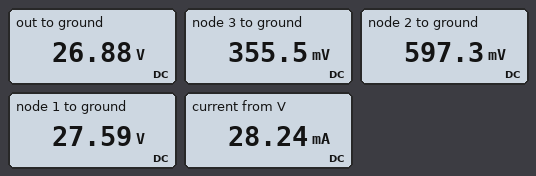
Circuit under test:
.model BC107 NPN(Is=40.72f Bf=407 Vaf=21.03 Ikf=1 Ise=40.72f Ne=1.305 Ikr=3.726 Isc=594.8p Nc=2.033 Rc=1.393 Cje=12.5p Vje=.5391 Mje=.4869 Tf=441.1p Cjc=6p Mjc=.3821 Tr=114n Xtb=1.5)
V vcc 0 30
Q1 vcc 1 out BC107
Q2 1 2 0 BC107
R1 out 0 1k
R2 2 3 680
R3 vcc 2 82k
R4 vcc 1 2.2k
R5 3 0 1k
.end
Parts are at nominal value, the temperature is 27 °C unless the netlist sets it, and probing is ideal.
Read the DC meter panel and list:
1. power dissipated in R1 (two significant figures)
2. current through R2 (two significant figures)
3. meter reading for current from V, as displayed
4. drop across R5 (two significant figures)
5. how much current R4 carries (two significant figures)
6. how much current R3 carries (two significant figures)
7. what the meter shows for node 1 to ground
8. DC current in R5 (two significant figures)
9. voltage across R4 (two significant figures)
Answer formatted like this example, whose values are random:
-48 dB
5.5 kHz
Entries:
720 mW
360 µA
28.24 mA
360 mV
1.1 mA
360 µA
27.59 V
360 µA
2.4 V
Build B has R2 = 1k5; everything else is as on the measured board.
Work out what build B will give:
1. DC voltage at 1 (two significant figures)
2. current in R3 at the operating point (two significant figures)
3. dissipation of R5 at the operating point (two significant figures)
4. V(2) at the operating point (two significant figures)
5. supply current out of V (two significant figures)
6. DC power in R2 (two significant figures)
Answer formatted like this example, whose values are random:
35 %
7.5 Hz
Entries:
200 mV
360 µA
76 µW
690 mV
14 mA
110 µW
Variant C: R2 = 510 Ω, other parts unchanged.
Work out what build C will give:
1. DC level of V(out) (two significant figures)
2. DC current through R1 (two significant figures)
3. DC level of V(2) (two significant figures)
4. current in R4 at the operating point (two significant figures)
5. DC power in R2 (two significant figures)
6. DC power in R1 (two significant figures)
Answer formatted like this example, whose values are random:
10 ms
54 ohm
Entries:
29 V
29 mA
540 mV
240 µA
66 µW
830 mW
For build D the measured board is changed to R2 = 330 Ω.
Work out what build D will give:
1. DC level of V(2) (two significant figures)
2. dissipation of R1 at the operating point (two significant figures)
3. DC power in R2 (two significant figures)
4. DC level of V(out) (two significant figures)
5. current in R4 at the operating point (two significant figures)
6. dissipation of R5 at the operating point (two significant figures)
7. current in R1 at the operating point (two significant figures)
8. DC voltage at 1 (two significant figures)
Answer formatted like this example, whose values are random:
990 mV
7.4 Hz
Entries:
480 mV
840 mW
43 µW
29 V
130 µA
130 µW
29 mA
30 V
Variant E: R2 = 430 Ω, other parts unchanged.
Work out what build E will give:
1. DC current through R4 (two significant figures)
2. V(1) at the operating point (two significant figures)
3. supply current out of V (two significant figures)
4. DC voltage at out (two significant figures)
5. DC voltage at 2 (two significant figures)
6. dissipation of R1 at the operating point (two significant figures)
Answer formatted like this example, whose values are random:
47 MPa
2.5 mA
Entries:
160 µA
30 V
29 mA
29 V
510 mV
840 mW
